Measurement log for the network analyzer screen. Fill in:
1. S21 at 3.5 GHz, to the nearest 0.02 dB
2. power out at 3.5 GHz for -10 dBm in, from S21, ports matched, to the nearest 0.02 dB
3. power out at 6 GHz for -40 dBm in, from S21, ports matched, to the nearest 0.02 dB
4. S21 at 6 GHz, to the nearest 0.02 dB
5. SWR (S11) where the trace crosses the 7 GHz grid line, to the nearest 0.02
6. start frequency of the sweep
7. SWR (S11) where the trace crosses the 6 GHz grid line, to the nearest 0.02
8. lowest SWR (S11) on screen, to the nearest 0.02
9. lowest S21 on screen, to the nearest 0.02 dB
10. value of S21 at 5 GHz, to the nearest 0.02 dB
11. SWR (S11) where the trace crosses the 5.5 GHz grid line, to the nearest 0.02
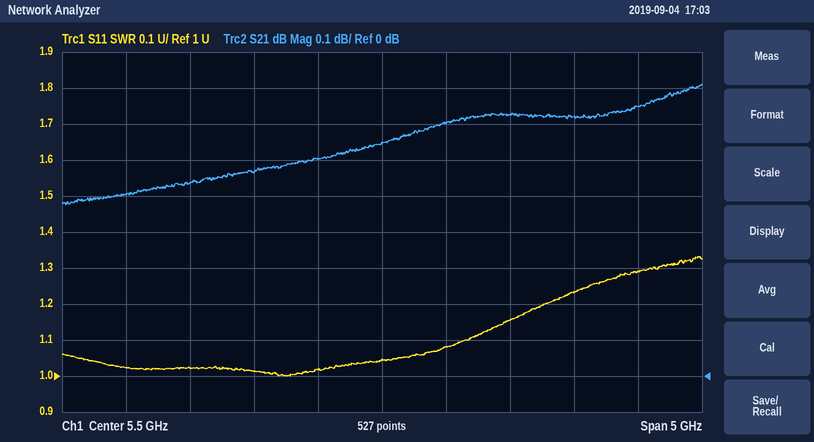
0.50 dB
-9.50 dBm
-39.30 dBm
0.70 dB
1.24
3 GHz
1.08
1.00
0.48 dB
0.60 dB
1.04
